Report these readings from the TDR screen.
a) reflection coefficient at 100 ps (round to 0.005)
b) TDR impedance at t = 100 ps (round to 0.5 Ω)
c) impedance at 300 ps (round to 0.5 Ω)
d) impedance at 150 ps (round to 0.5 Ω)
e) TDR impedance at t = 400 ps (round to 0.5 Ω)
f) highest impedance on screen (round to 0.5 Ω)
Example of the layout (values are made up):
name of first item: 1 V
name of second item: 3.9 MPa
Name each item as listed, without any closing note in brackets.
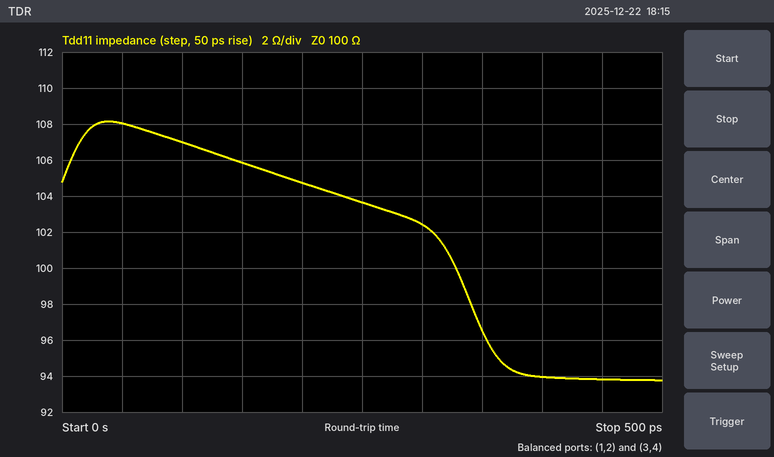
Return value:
reflection coefficient at 100 ps: +0.035
TDR impedance at t = 100 ps: 107.0 Ω
impedance at 300 ps: 102.5 Ω
impedance at 150 ps: 106.0 Ω
TDR impedance at t = 400 ps: 94.0 Ω
highest impedance on screen: 108.0 Ω
